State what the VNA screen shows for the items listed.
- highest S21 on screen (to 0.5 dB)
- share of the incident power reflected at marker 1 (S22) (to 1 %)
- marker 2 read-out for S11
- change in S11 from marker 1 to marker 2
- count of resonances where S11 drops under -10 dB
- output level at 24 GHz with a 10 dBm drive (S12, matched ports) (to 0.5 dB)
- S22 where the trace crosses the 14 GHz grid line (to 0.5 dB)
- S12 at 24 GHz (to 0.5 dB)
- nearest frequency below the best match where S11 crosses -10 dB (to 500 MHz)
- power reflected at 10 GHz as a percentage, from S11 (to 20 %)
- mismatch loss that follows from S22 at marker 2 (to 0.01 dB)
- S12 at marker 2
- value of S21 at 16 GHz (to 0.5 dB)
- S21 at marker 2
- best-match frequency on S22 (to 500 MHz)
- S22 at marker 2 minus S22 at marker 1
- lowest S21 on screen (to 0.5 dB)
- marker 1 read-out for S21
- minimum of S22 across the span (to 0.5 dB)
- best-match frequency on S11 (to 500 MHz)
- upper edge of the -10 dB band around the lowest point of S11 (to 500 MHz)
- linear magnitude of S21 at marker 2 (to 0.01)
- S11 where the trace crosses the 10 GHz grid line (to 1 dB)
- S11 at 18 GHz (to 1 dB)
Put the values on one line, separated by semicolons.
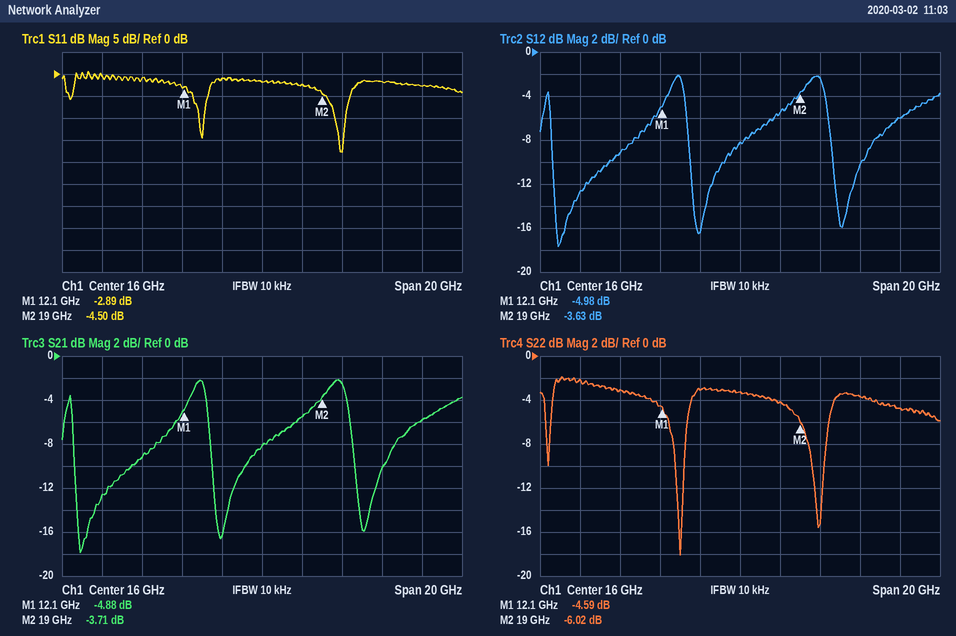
-2.0 dB; 35 %; -4.50 dB; -1.61 dB; 2; 4.0 dBm; -3.0 dB; -6.0 dB; 19.5 GHz; 80 %; 1.25 dB; -3.63 dB; -8.0 dB; -3.71 dB; 13.0 GHz; -1.43 dB; -18.0 dB; -4.88 dB; -18.0 dB; 20.0 GHz; 20.0 GHz; 0.65; -1 dB; -2 dB
